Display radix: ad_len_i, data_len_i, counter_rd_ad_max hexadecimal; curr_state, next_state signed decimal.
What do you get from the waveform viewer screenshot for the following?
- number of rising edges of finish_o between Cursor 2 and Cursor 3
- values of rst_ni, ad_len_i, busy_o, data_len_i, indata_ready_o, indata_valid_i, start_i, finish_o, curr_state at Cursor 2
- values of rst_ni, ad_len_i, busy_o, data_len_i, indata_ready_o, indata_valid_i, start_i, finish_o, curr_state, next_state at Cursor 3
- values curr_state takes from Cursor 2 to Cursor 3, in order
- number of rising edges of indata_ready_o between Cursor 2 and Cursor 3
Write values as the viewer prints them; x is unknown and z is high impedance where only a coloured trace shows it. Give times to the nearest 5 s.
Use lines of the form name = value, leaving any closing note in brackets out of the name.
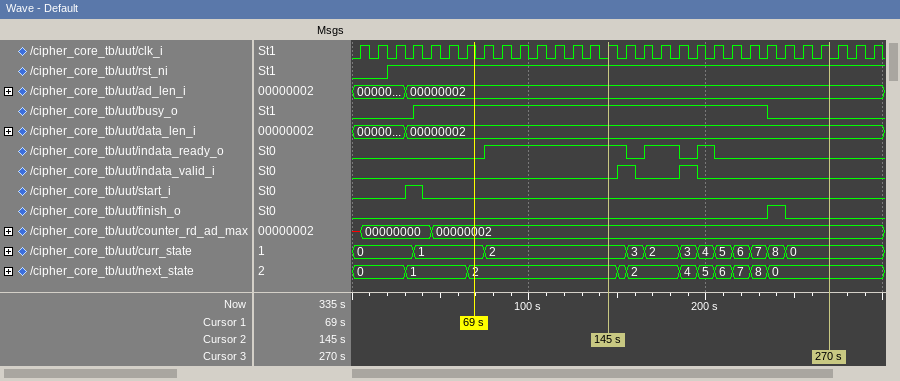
number of rising edges of finish_o between Cursor 2 and Cursor 3 = 1
values of rst_ni, ad_len_i, busy_o, data_len_i, indata_ready_o, indata_valid_i, start_i, finish_o, curr_state at Cursor 2 = rst_ni=1, ad_len_i=00000002, busy_o=1, data_len_i=00000002, indata_ready_o=1, indata_valid_i=0, start_i=0, finish_o=0, curr_state=2
values of rst_ni, ad_len_i, busy_o, data_len_i, indata_ready_o, indata_valid_i, start_i, finish_o, curr_state, next_state at Cursor 3 = rst_ni=1, ad_len_i=00000002, busy_o=0, data_len_i=00000002, indata_ready_o=0, indata_valid_i=0, start_i=0, finish_o=0, curr_state=0, next_state=0
values curr_state takes from Cursor 2 to Cursor 3, in order = 2, 3, 2, 3, 4, 5, 6, 7, 8, 0
number of rising edges of indata_ready_o between Cursor 2 and Cursor 3 = 2
